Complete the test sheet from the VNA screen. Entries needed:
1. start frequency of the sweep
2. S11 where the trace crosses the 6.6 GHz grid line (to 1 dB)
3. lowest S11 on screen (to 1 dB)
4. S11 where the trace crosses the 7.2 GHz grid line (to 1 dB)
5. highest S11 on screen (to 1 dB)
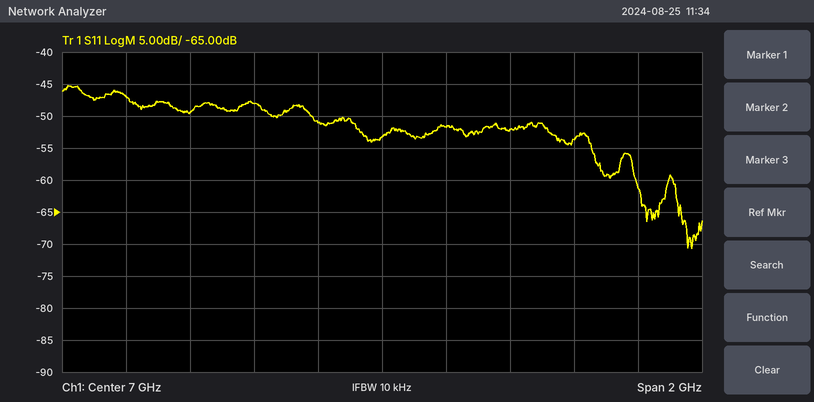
6 GHz
-48 dB
-71 dB
-52 dB
-45 dB
